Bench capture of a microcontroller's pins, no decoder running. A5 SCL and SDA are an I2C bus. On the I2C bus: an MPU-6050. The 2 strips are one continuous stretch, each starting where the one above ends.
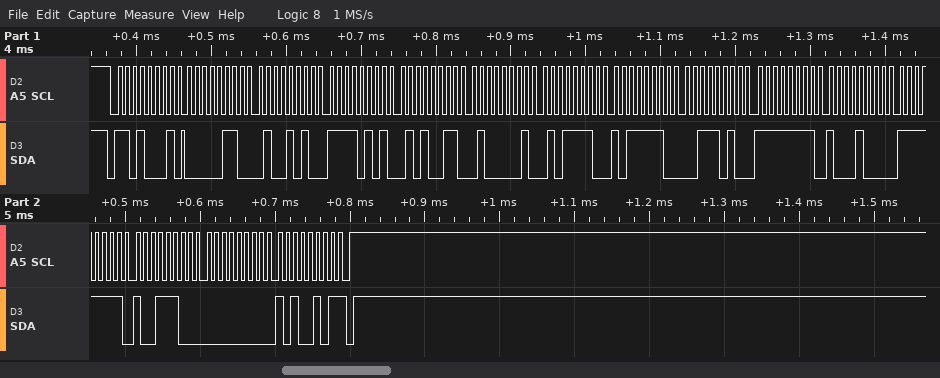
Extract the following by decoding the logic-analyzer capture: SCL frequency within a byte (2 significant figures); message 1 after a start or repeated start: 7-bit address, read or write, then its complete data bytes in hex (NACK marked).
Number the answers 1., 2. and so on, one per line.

1. 100 kHz
2. 0x68 read: 06 4A F5 53 41 5E BE 3A FF 88 FF 9C 00 A5 NACK
